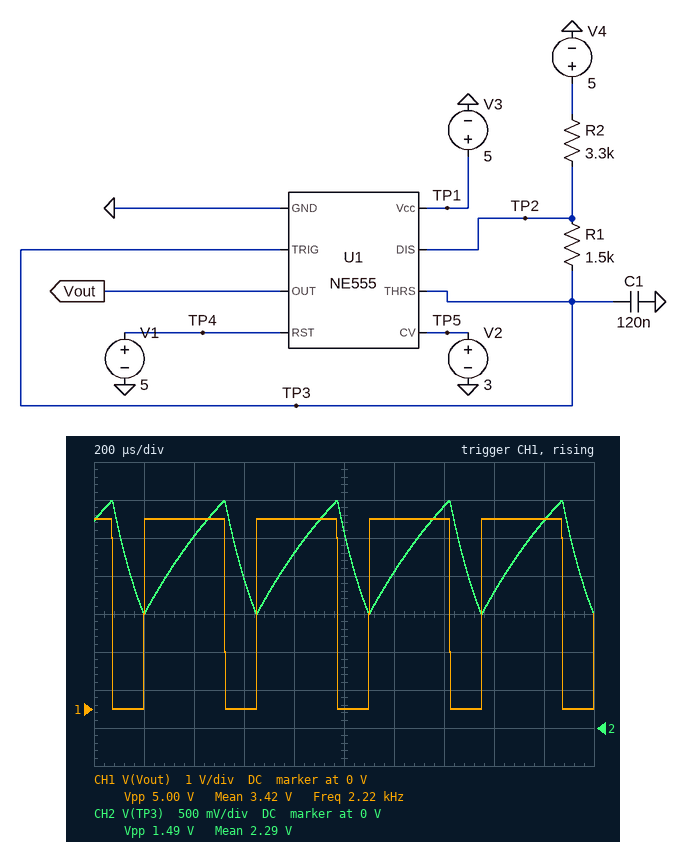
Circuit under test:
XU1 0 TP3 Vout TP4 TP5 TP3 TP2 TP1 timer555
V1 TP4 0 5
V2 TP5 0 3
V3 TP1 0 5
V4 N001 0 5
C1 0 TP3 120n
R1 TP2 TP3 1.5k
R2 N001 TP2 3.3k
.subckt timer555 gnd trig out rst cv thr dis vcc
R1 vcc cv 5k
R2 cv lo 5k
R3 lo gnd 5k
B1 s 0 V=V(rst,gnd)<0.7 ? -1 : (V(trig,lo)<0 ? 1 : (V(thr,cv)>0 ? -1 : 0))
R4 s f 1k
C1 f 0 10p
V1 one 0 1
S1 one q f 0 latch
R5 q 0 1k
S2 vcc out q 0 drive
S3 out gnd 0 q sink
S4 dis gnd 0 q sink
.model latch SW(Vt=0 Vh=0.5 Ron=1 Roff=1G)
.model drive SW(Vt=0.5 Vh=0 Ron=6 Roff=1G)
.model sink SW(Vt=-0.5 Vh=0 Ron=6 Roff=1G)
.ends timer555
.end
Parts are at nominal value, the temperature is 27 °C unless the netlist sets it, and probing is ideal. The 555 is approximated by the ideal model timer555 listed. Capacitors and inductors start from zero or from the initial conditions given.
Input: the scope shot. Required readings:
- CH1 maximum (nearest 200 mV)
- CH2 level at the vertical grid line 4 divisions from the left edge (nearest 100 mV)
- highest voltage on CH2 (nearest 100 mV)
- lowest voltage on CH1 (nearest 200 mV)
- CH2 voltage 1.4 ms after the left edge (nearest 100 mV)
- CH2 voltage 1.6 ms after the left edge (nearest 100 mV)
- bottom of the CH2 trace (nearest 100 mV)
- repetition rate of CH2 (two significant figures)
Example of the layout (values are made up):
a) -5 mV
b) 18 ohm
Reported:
a) 5.0 V
b) 2.3 V
c) 3.0 V
d) 0 V
e) 2.9 V
f) 1.8 V
g) 1.5 V
h) 2.2 kHz
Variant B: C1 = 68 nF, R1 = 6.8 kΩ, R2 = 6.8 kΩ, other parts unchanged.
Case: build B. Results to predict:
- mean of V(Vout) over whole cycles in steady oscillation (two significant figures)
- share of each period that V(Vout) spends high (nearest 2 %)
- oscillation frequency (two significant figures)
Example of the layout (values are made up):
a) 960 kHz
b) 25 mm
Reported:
a) 3.1 V
b) 62 %
c) 1.2 kHz
